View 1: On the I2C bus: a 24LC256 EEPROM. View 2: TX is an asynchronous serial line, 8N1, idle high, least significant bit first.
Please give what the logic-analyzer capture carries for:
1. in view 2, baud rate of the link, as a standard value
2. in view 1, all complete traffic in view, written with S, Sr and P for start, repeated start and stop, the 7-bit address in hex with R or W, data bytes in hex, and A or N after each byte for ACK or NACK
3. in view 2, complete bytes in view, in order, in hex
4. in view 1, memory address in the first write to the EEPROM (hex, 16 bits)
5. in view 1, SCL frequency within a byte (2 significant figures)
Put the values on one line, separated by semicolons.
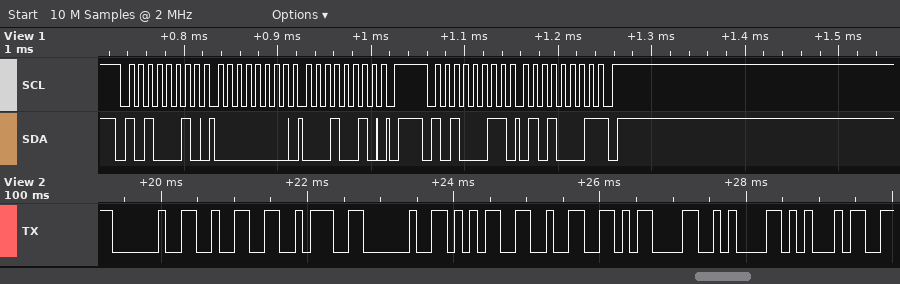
9600 baud; S 51W A 00 A 12 A P S 51R A 51 N P; 20 32 3A 20 35 32 0D 0A 45; 0x0012; 100 kHz
